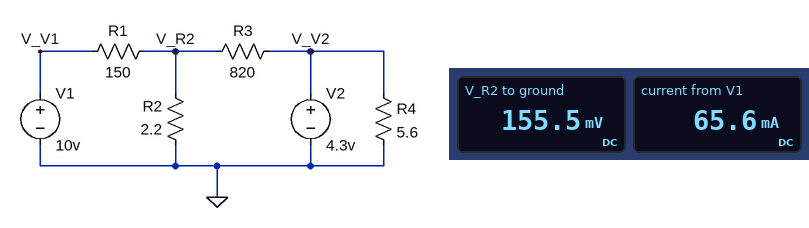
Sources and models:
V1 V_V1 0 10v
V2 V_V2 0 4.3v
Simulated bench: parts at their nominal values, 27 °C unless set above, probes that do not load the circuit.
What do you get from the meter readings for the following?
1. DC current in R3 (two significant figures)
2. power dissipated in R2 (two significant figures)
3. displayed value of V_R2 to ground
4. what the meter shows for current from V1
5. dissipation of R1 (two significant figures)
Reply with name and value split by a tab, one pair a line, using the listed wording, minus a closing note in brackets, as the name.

DC current in R3	5.1 mA
power dissipated in R2	11 mW
displayed value of V_R2 to ground	155.5 mV
what the meter shows for current from V1	65.6 mA
dissipation of R1	650 mW
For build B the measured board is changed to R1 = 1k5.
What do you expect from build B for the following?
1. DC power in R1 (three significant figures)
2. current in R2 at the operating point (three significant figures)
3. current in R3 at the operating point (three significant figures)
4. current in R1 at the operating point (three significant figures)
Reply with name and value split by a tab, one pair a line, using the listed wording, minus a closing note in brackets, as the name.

DC power in R1	66.3 mW
current in R2 at the operating point	11.9 mA
current in R3 at the operating point	5.21 mA
current in R1 at the operating point	6.65 mA
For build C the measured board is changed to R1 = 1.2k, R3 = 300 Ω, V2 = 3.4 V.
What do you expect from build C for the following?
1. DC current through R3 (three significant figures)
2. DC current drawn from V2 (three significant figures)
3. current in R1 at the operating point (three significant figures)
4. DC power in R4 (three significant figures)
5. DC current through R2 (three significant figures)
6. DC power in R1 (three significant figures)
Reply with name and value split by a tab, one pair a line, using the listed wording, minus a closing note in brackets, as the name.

DC current through R3	11.2 mA
DC current drawn from V2	618 mA
current in R1 at the operating point	8.30 mA
DC power in R4	2.06 W
DC current through R2	19.5 mA
DC power in R1	82.6 mW
